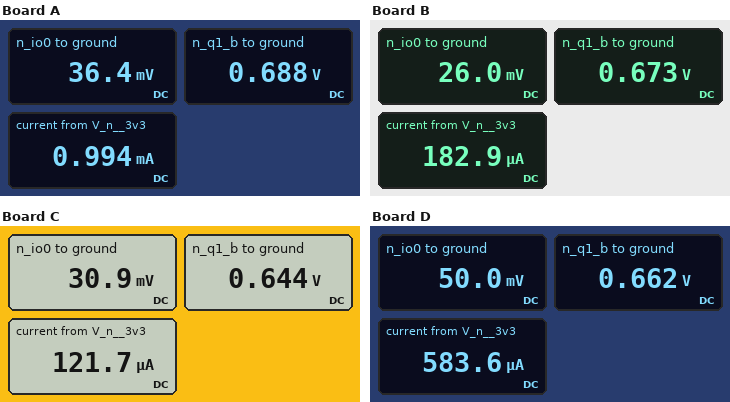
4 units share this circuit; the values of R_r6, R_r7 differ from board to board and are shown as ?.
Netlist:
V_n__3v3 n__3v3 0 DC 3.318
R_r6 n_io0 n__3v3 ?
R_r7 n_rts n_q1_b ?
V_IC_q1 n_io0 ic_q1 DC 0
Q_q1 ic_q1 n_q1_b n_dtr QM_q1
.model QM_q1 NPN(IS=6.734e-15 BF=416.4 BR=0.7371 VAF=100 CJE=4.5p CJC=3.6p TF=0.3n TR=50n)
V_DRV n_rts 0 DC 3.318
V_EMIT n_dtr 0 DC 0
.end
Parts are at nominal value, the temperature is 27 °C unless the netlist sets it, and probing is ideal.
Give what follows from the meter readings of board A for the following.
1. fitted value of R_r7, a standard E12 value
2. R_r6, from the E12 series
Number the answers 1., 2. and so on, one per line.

1. 3.3 kΩ
2. 3.3 kΩ
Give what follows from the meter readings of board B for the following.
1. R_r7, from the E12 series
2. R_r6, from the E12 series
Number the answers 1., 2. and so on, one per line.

1. 3.9 kΩ
2. 18 kΩ
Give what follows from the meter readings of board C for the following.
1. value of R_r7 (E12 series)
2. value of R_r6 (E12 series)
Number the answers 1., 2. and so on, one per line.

1. 15 kΩ
2. 27 kΩ
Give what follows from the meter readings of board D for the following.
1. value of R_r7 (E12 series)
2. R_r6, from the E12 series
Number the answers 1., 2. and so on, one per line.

1. 15 kΩ
2. 5.6 kΩ
